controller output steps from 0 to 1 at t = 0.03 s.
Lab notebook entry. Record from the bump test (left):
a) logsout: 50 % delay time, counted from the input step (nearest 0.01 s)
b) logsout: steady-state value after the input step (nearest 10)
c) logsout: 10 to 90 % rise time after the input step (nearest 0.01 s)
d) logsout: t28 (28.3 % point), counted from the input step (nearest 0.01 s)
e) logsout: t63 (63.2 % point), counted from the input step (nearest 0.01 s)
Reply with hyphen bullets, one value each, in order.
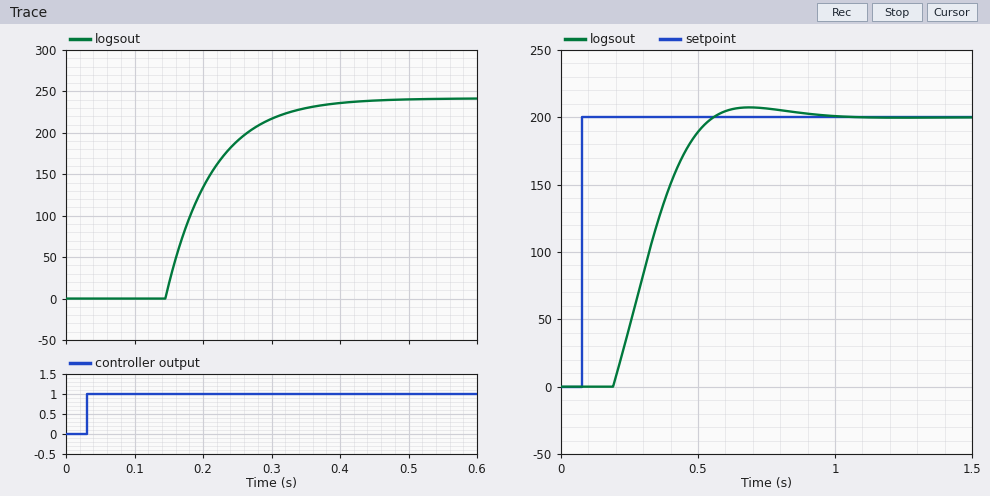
- 0.16 s
- 240
- 0.15 s
- 0.14 s
- 0.18 s
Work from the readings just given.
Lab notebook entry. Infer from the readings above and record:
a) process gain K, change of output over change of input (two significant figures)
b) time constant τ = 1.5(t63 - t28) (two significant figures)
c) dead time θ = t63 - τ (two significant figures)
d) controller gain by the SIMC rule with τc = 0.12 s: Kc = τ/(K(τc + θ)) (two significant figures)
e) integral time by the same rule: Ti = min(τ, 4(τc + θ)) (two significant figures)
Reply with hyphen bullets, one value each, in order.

- 240
- 0.060 s
- 0.12 s
- 0.0010
- 0.060 s
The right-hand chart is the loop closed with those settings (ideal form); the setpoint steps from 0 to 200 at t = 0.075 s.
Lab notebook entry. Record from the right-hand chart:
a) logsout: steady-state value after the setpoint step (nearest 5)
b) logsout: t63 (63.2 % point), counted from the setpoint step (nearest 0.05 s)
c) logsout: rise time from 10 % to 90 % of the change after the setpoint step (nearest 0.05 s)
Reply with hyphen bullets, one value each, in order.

- 200
- 0.30 s
- 0.25 s
